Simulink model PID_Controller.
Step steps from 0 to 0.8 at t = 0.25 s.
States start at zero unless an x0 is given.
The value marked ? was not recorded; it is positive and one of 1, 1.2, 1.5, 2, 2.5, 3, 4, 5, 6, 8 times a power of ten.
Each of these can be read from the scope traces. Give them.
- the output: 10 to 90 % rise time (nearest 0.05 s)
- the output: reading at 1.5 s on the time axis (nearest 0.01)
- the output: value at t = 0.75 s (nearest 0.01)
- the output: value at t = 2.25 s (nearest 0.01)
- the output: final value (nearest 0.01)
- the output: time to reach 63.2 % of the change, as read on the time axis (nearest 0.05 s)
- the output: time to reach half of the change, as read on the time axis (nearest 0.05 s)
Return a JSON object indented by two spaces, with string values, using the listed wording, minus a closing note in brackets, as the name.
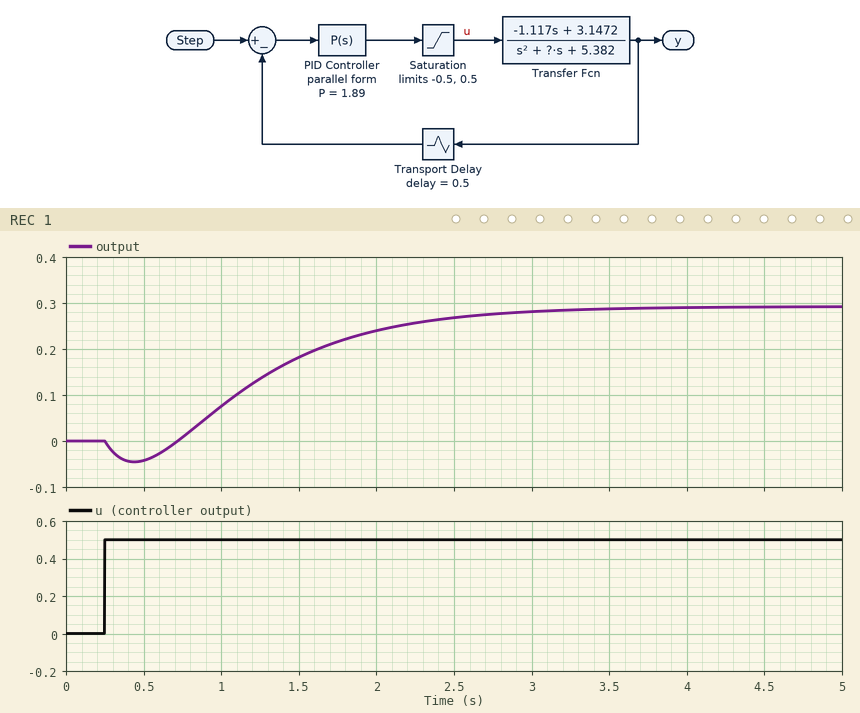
{
  "the output: 10 to 90 % rise time": "1.55 s",
  "the output: reading at 1.5 s on the time axis": "0.18",
  "the output: value at t = 0.75 s": "0.01",
  "the output: value at t = 2.25 s": "0.26",
  "the output: final value": "0.29",
  "the output: time to reach 63.2 % of the change, as read on the time axis": "1.50 s",
  "the output: time to reach half of the change, as read on the time axis": "1.30 s"
}
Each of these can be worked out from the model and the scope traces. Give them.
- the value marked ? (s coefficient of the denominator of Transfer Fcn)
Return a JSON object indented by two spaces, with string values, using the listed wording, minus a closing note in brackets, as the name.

{
  "the value marked ?": "5"
}
